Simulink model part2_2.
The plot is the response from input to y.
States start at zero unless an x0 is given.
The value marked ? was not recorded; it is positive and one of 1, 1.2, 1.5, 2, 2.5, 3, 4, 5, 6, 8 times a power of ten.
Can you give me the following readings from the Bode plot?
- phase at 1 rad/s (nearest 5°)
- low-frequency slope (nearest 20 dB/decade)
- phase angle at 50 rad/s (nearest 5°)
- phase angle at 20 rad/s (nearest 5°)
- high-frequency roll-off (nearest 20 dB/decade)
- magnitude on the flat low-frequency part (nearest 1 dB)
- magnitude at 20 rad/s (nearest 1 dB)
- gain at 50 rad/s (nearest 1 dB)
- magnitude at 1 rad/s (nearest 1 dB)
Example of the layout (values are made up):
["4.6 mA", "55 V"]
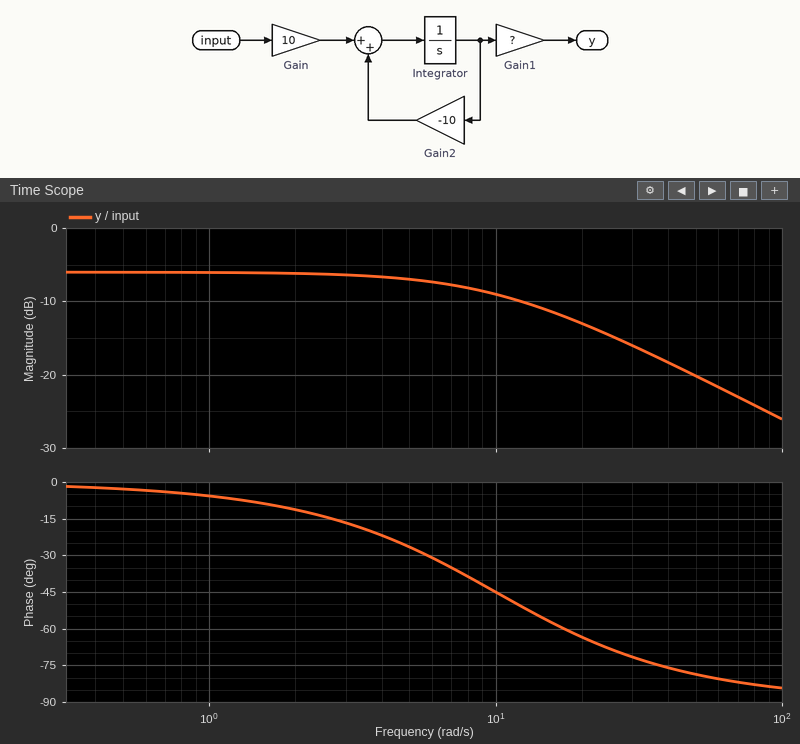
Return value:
["-5°", "0 dB/decade", "-80°", "-65°", "-20 dB/decade", "-6 dB", "-13 dB", "-20 dB", "-6 dB"]
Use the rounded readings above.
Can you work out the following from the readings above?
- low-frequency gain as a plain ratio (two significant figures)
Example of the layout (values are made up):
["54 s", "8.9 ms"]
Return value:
["0.50"]
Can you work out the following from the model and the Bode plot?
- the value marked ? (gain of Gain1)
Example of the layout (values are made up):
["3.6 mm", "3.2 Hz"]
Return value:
["0.5"]
